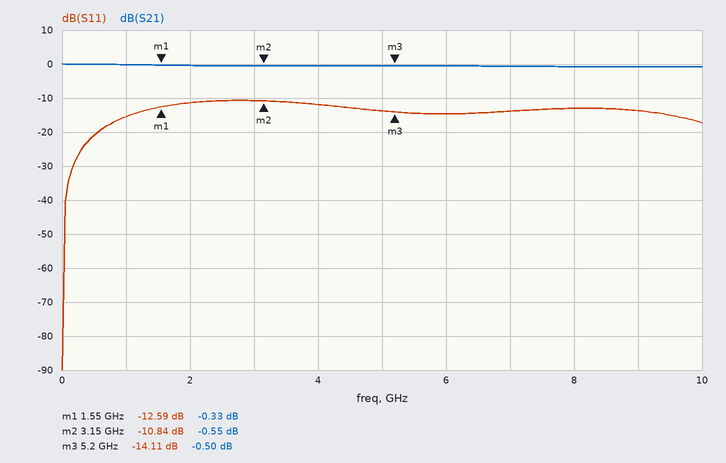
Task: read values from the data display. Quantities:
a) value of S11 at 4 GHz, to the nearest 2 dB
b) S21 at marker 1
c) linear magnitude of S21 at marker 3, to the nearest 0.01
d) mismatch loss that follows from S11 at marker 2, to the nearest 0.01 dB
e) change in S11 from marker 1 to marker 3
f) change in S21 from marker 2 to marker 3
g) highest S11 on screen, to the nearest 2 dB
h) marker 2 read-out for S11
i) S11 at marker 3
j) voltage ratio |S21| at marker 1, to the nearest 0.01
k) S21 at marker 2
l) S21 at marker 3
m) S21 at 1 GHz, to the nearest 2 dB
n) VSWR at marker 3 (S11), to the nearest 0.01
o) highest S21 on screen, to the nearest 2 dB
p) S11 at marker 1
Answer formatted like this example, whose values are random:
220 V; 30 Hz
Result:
-12 dB; -0.33 dB; 0.94; 0.37 dB; -1.52 dB; 0.05 dB; -10 dB; -10.84 dB; -14.11 dB; 0.96; -0.55 dB; -0.50 dB; 0 dB; 1.49; 0 dB; -12.59 dB
